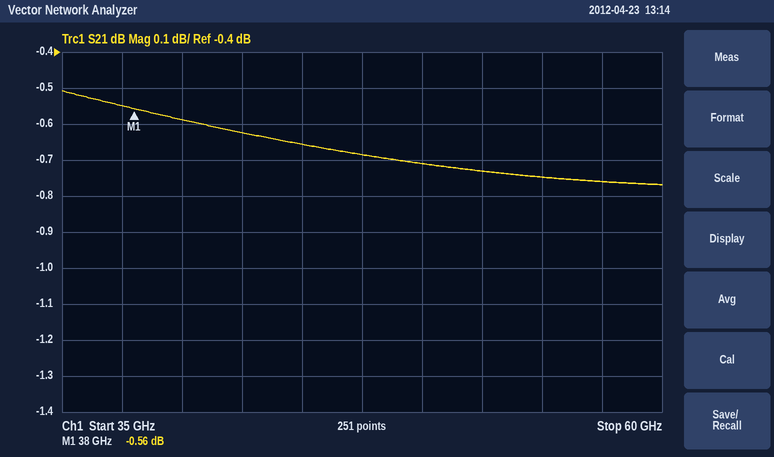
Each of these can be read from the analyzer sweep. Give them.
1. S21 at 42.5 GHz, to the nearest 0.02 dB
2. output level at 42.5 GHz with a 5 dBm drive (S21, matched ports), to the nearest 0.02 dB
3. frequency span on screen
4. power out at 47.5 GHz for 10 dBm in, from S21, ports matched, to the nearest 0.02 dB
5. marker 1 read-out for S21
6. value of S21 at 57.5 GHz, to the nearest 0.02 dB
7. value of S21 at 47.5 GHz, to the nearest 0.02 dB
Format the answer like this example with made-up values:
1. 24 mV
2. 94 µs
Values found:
1. -0.62 dB
2. 4.38 dBm
3. 25 GHz
4. 9.32 dBm
5. -0.56 dB
6. -0.76 dB
7. -0.68 dB
